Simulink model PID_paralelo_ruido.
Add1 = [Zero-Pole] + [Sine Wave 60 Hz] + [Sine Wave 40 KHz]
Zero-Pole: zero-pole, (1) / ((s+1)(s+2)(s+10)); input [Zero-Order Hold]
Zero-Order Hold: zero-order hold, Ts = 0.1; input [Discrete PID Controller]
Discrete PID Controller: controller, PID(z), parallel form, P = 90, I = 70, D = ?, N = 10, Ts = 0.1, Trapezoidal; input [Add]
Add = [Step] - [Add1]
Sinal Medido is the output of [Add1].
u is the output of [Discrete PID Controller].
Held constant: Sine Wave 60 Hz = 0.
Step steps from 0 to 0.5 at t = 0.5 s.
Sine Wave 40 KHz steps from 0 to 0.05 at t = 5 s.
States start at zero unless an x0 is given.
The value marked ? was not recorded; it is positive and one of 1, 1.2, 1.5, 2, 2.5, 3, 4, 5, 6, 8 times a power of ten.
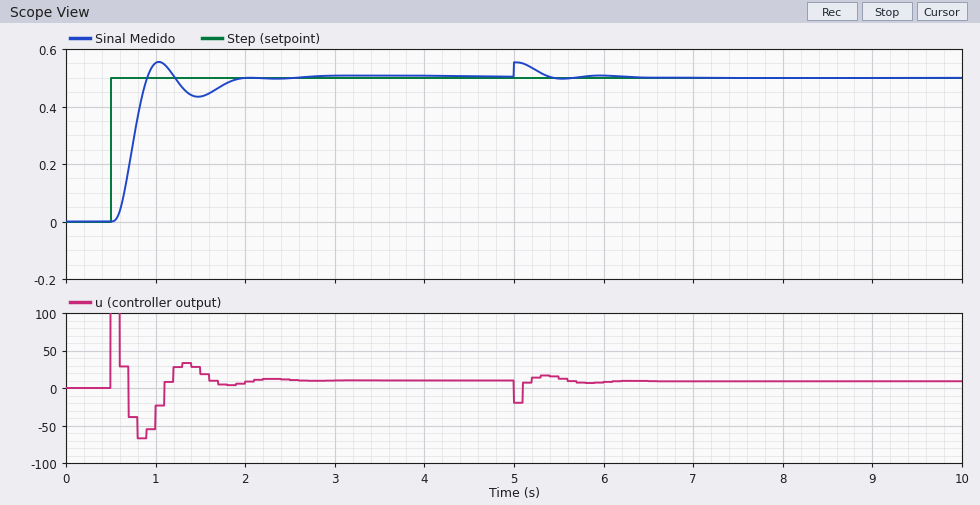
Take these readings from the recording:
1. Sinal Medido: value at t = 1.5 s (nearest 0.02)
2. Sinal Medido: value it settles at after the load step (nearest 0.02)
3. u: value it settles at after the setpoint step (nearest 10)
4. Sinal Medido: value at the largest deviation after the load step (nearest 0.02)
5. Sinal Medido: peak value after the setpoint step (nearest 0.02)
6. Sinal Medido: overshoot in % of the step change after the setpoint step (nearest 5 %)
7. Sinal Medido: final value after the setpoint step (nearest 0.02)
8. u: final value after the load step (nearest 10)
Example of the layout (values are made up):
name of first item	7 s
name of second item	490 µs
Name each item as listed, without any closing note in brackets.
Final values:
Sinal Medido: value at t = 1.5 s	0.44
Sinal Medido: value it settles at after the load step	0.50
u: value it settles at after the setpoint step	10
Sinal Medido: value at the largest deviation after the load step	0.56
Sinal Medido: peak value after the setpoint step	0.56
Sinal Medido: overshoot in % of the step change after the setpoint step	10 %
Sinal Medido: final value after the setpoint step	0.50
u: final value after the load step	10
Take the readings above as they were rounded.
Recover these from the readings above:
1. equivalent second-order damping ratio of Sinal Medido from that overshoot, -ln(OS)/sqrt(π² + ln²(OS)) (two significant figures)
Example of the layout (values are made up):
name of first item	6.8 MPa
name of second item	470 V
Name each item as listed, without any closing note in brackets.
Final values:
equivalent second-order damping ratio of Sinal Medido from that overshoot, -ln(OS)/sqrt(π² + ln²(OS))	0.59
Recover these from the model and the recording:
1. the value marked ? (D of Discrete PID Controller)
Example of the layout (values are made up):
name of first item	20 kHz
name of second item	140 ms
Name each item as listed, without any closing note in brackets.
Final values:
the value marked ?	50
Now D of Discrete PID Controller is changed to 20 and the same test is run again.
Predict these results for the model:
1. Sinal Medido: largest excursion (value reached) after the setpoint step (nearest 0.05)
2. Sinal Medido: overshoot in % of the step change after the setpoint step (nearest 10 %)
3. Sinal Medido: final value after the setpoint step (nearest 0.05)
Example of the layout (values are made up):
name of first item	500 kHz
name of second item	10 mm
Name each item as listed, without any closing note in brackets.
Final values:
Sinal Medido: largest excursion (value reached) after the setpoint step	0.60
Sinal Medido: overshoot in % of the step change after the setpoint step	20 %
Sinal Medido: final value after the setpoint step	0.50
